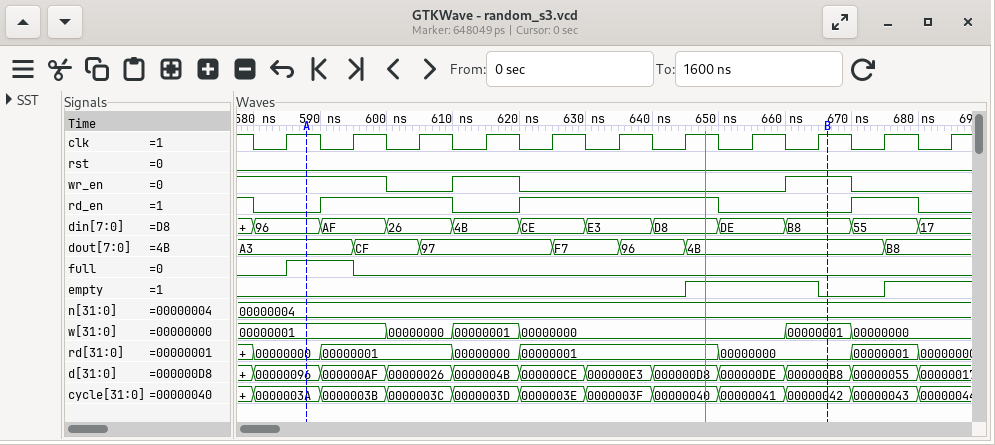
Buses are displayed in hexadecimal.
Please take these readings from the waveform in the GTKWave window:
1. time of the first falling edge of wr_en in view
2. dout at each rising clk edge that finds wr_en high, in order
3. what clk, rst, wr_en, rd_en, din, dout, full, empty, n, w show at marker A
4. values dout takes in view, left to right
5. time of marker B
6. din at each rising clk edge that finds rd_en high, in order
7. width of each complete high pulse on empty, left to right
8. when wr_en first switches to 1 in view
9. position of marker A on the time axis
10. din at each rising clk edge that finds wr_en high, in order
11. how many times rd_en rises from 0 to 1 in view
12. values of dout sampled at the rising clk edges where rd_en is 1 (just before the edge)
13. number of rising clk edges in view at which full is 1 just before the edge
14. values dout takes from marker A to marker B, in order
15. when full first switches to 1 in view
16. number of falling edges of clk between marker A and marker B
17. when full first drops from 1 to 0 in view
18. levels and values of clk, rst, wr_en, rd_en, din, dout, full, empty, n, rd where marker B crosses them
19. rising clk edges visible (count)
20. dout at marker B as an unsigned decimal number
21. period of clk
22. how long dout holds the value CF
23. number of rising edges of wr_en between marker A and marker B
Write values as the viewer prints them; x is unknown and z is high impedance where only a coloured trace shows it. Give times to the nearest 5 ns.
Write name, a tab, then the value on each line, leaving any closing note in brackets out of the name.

time of the first falling edge of wr_en in view	600 ns
dout at each rising clk edge that finds wr_en high, in order	A3, A3, 97, 4B
what clk, rst, wr_en, rd_en, din, dout, full, empty, n, w show at marker A	clk=1, rst=0, wr_en=1, rd_en=0, din=96, dout=A3, full=1, empty=0, n=00000004, w=00000001
values dout takes in view, left to right	A3, CF, 97, F7, 96, 4B, B8
time of marker B	665 ns
din at each rising clk edge that finds rd_en high, in order	AF, 26, CE, E3, D8, 55
width of each complete high pulse on empty, left to right	20 ns
when wr_en first switches to 1 in view	610 ns
position of marker A on the time axis	590 ns
din at each rising clk edge that finds wr_en high, in order	96, AF, 4B, B8
how many times rd_en rises from 0 to 1 in view	3
values of dout sampled at the rising clk edges where rd_en is 1	A3, CF, 97, F7, 96, 4B
number of rising clk edges in view at which full is 1 just before the edge	1
values dout takes from marker A to marker B, in order	A3, CF, 97, F7, 96, 4B
when full first switches to 1 in view	585 ns
number of falling edges of clk between marker A and marker B	8
when full first drops from 1 to 0 in view	595 ns
levels and values of clk, rst, wr_en, rd_en, din, dout, full, empty, n, rd where marker B crosses them	clk=1, rst=0, wr_en=1, rd_en=0, din=B8, dout=4B, full=0, empty=0, n=00000004, rd=00000000
rising clk edges visible	11
dout at marker B as an unsigned decimal number	75
period of clk	10 ns
how long dout holds the value CF	10 ns
number of rising edges of wr_en between marker A and marker B	2
